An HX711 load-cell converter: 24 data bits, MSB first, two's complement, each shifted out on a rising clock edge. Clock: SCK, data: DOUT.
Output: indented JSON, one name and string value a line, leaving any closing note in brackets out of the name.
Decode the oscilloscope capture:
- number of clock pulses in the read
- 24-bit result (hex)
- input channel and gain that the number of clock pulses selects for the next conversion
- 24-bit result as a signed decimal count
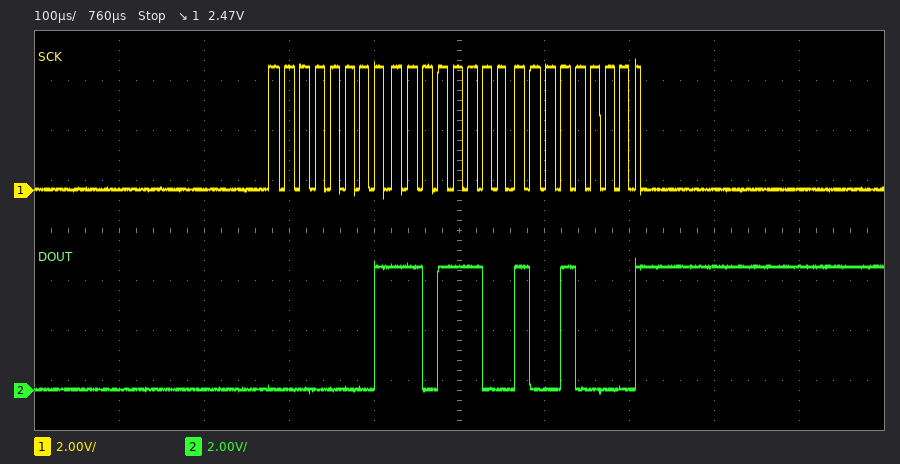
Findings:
{
  "number of clock pulses in the read": "25",
  "24-bit result": "0x01DC90",
  "input channel and gain that the number of clock pulses selects for the next conversion": "channel A, gain 128",
  "24-bit result as a signed decimal count": "122000"
}
